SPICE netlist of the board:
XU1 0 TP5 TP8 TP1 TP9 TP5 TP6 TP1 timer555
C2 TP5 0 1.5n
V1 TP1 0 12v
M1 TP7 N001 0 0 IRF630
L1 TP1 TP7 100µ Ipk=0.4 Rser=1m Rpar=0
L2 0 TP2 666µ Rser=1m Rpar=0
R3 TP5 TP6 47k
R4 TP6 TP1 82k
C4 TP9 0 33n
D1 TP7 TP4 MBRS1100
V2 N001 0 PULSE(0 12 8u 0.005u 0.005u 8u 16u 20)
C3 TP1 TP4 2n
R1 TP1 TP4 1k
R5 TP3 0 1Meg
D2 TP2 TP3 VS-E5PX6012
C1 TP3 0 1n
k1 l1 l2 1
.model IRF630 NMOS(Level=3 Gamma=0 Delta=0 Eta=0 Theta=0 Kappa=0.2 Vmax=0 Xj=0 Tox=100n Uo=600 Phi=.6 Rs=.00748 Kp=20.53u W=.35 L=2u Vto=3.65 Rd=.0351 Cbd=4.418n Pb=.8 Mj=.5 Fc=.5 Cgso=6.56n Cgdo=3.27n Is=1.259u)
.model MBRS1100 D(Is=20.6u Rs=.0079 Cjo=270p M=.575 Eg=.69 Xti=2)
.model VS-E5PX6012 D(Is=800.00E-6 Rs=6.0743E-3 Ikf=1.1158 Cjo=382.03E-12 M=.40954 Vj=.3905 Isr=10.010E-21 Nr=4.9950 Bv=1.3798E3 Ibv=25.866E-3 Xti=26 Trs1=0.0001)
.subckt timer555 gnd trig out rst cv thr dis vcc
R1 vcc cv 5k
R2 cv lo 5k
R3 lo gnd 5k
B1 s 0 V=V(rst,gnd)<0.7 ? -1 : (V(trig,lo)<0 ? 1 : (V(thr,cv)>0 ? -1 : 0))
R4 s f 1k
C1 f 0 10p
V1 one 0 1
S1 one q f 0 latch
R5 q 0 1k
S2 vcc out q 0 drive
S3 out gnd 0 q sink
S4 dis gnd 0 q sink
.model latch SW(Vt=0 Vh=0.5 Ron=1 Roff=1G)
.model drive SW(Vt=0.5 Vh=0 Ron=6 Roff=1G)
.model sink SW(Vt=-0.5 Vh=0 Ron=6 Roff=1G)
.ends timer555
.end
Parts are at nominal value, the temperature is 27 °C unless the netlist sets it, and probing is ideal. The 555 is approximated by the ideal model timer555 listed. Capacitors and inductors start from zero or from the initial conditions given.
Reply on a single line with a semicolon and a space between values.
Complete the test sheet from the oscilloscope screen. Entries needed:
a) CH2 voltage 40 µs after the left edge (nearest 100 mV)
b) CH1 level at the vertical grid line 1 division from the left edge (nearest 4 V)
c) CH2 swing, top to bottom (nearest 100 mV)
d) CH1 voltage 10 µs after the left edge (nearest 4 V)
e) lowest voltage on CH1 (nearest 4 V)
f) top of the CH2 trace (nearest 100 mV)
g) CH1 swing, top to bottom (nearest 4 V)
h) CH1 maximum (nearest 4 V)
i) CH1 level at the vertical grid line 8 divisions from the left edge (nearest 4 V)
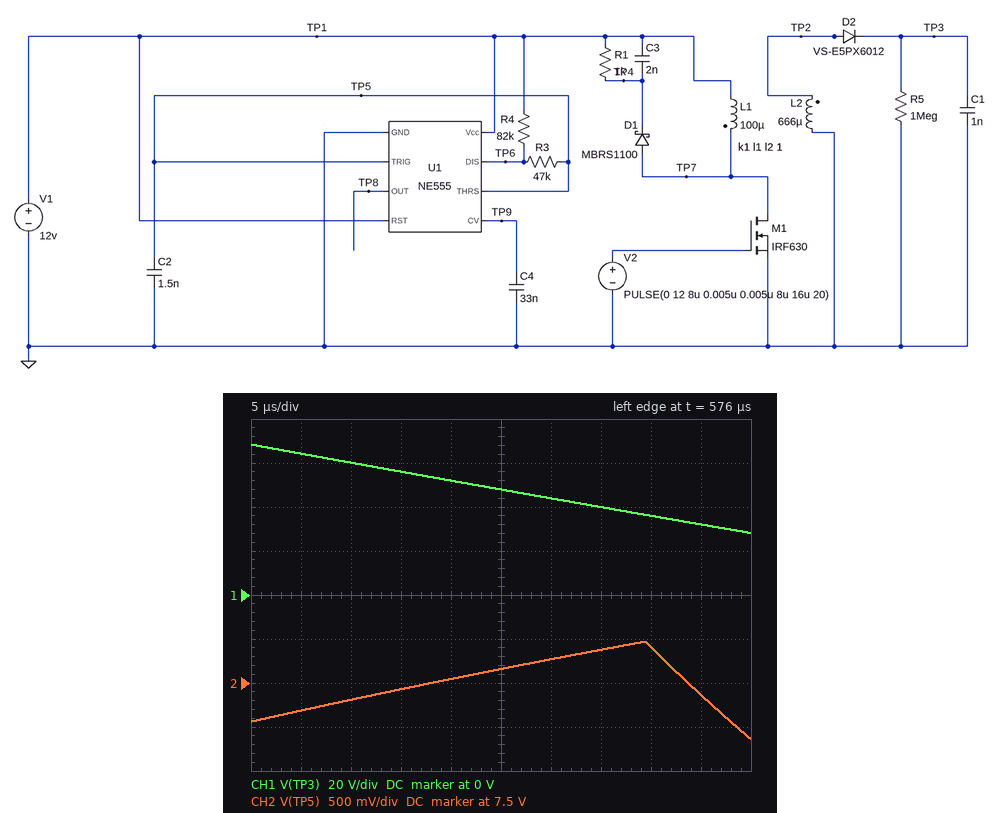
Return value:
7.9 V; 64 V; 1.1 V; 60 V; 28 V; 8.0 V; 40 V; 68 V; 36 V
